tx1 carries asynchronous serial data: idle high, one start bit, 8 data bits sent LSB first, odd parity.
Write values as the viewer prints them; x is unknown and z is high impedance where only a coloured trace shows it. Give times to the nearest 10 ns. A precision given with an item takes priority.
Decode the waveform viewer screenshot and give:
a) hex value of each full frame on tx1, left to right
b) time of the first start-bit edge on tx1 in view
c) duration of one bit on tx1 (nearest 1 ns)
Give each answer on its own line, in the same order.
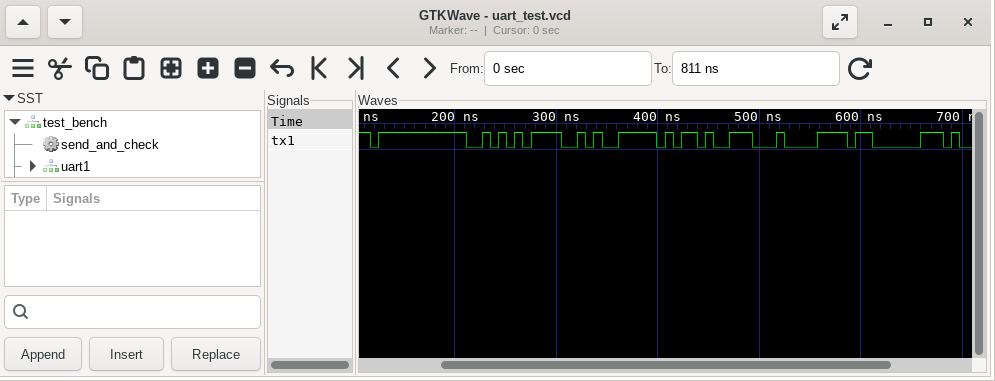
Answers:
FF, AA, CA, 2D, 84, 03
120 ns
8 ns
